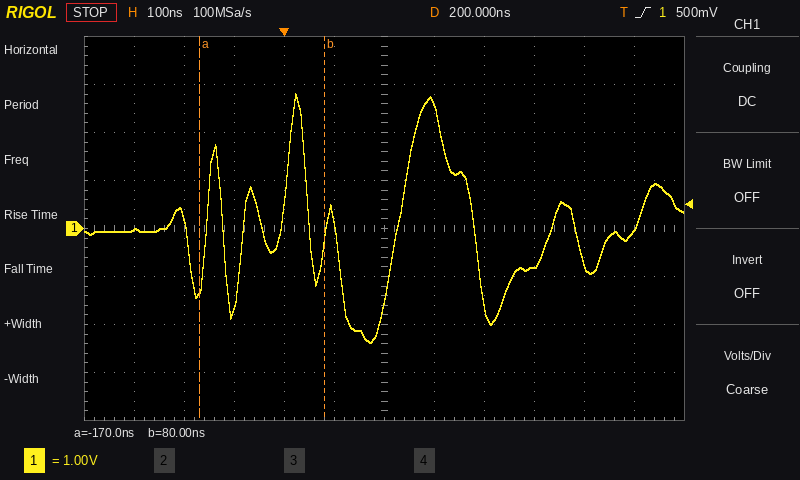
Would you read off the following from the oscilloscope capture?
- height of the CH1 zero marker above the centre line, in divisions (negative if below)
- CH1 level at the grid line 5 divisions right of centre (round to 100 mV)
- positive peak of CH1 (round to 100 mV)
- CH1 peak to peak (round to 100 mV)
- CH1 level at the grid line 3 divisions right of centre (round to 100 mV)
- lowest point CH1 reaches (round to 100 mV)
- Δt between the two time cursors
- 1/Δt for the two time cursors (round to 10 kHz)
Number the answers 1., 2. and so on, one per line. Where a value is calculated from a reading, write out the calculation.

1. 0.0 div
2. 0.0 V
3. 2.8 V
4. 2.8 V − (-2.4 V) = 5.2 V
5. -800 mV
6. -2.4 V
7. 80 ns − (-170 ns) = 250 ns
8. 1 / 250 ns ≈ 4.00 MHz
